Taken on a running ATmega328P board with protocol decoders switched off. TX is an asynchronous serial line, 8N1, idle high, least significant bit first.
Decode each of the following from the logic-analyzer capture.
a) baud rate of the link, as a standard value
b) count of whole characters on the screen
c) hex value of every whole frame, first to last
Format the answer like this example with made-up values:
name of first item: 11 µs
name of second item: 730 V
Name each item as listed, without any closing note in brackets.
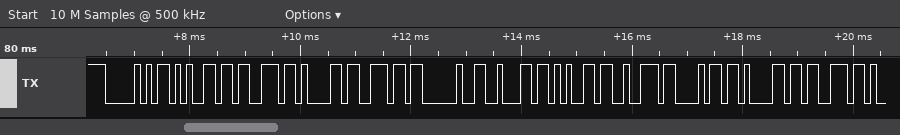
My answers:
baud rate of the link, as a standard value: 9600 baud
count of whole characters on the screen: 12
hex value of every whole frame, first to last: 0x50 0x65 0x73 0x61 0x6E 0x20 0x62 0x65 0x72 0x68 0x61 0x73
